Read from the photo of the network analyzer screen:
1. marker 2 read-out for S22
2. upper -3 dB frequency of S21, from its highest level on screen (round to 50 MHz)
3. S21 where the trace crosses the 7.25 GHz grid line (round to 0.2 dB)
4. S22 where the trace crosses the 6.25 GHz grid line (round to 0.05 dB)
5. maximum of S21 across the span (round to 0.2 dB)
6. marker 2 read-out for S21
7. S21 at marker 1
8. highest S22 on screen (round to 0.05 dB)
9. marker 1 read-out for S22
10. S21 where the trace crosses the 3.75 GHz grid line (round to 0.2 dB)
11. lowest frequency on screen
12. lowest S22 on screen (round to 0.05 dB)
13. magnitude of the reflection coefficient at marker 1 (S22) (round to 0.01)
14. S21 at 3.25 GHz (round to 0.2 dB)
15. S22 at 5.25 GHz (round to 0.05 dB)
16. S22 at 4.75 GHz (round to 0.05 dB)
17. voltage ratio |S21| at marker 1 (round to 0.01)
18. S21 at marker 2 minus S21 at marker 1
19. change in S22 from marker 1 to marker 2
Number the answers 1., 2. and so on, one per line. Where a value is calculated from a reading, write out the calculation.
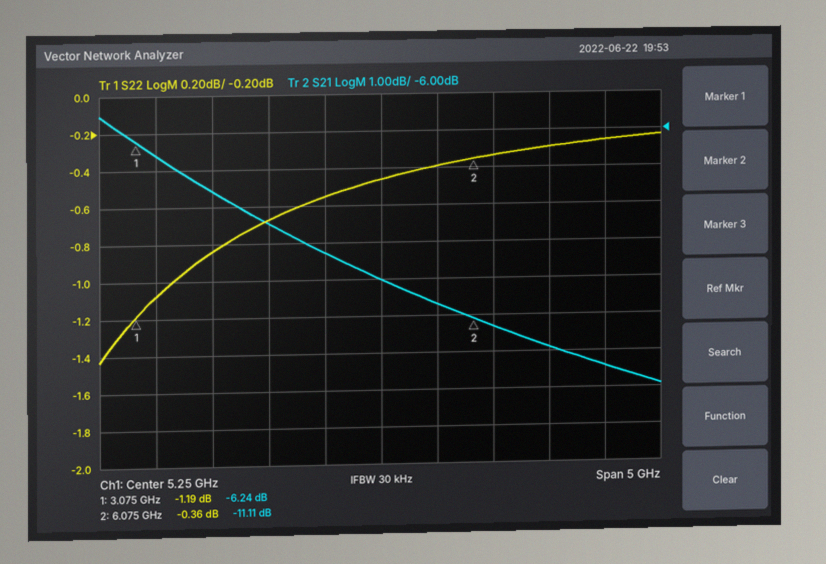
1. -0.36 dB
2. 4.30 GHz
3. -12.4 dB
4. -0.35 dB
5. -5.6 dB
6. -11.11 dB
7. -6.24 dB
8. -0.25 dB
9. -1.19 dB
10. -7.6 dB
11. 2.75 GHz
12. -1.45 dB
13. 10^(-1.19/20) ≈ 0.87
14. -6.6 dB
15. -0.45 dB
16. -0.55 dB
17. 10^(-6.24/20) ≈ 0.49
18. -11.11 − (-6.24) = -4.87 dB
19. -0.36 − (-1.19) = 0.83 dB
